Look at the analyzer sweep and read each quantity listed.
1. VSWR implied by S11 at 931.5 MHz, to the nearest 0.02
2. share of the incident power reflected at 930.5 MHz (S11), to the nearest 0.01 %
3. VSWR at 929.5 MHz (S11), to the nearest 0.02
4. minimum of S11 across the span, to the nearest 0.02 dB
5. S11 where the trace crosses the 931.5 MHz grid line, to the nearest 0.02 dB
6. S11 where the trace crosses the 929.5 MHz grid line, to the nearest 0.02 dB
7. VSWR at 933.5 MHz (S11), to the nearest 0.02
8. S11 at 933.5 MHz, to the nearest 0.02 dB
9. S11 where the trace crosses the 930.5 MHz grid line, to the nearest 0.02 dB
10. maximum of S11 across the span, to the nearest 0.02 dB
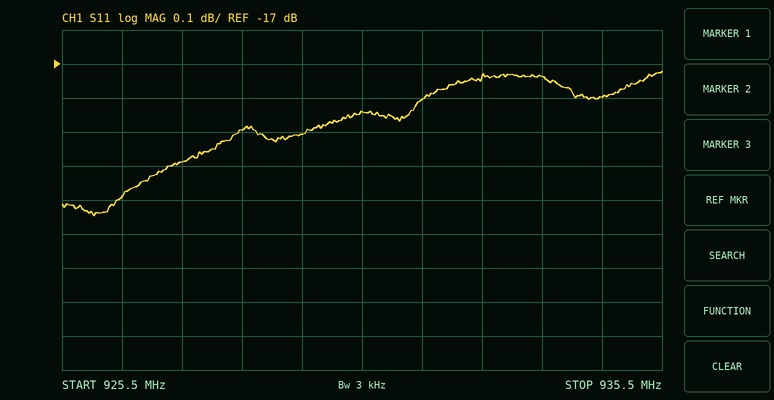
1.32
1.93 %
1.32
-17.44 dB
-17.10 dB
-17.20 dB
1.32
-17.04 dB
-17.14 dB
-17.02 dB
